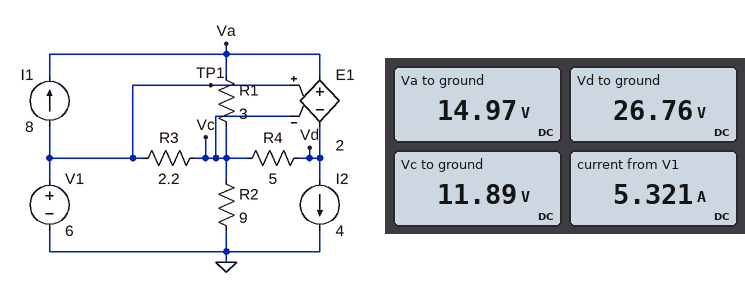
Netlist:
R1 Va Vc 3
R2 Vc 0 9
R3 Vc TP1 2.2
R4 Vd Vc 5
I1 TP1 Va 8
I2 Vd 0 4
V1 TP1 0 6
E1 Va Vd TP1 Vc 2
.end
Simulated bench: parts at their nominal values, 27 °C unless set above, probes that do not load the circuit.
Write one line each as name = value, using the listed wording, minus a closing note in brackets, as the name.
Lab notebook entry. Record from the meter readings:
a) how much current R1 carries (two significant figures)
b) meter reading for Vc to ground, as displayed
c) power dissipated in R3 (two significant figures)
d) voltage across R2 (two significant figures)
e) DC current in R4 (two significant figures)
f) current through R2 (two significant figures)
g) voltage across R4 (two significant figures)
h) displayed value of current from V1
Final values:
how much current R1 carries = 1.0 A
meter reading for Vc to ground, as displayed = 11.89 V
power dissipated in R3 = 16 W
voltage across R2 = 12 V
DC current in R4 = 3.0 A
current through R2 = 1.3 A
voltage across R4 = 15 V
displayed value of current from V1 = 5.321 A
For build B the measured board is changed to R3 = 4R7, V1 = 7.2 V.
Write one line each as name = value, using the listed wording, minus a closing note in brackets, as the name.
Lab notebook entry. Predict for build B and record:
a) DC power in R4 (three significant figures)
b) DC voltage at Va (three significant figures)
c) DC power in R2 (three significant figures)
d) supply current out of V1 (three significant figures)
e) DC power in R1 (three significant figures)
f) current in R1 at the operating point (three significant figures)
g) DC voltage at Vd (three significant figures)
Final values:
DC power in R4 = 78.8 W
DC voltage at Va = 17.2 V
DC power in R2 = 32.4 W
supply current out of V1 = 5.90 A
DC power in R1 = 2.69 mW
current in R1 at the operating point = 29.9 mA
DC voltage at Vd = 36.9 V
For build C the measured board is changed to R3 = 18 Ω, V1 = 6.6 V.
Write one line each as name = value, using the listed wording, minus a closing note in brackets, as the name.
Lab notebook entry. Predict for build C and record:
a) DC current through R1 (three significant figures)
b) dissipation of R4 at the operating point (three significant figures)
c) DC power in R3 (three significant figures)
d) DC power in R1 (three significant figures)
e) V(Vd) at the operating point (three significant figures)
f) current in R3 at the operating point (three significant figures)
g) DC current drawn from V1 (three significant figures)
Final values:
DC current through R1 = 2.40 A
dissipation of R4 at the operating point = 205 W
DC power in R3 = 21.3 W
DC power in R1 = 17.3 W
V(Vd) at the operating point = 58.2 V
current in R3 at the operating point = 1.09 A
DC current drawn from V1 = 6.91 A
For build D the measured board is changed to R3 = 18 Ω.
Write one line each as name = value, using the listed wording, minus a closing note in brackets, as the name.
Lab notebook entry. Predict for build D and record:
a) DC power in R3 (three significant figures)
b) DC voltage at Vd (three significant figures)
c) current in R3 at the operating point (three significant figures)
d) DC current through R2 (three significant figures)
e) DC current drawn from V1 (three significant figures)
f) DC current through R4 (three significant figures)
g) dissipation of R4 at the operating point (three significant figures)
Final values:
DC power in R3 = 22.2 W
DC voltage at Vd = 58.5 V
current in R3 at the operating point = 1.11 A
DC current through R2 = 2.89 A
DC current drawn from V1 = 6.89 A
DC current through R4 = 6.50 A
dissipation of R4 at the operating point = 211 W
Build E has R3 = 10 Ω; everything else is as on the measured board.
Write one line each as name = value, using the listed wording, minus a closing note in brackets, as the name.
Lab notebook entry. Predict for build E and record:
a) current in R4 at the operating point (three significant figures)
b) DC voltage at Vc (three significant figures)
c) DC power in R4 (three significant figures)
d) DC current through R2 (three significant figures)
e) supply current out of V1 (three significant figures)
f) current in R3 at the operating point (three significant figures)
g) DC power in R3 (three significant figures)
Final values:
current in R4 at the operating point = 5.45 A
DC voltage at Vc = 21.8 V
DC power in R4 = 148 W
DC current through R2 = 2.42 A
supply current out of V1 = 6.42 A
current in R3 at the operating point = 1.58 A
DC power in R3 = 24.9 W
